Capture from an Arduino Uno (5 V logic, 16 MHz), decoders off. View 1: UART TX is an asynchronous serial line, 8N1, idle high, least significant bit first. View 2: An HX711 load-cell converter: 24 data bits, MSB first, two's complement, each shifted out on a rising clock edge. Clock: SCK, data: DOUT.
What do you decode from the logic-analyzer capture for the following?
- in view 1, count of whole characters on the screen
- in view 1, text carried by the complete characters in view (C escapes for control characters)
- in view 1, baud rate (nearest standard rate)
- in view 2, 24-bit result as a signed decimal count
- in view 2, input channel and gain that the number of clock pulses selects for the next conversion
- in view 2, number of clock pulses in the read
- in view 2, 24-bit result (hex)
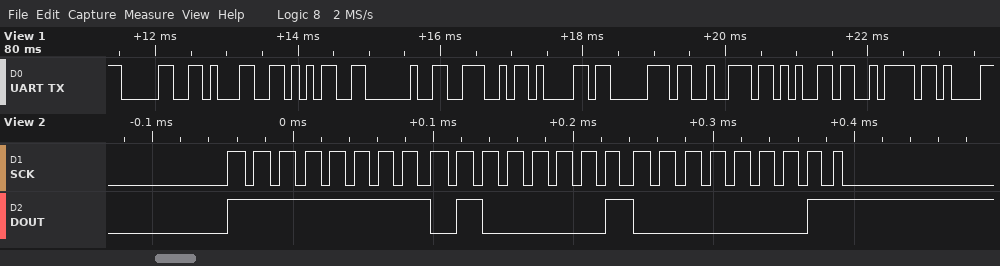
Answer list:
10
"015 Naprez"
9600 baud
-48895
channel A, gain 128
25
0xFF4101
